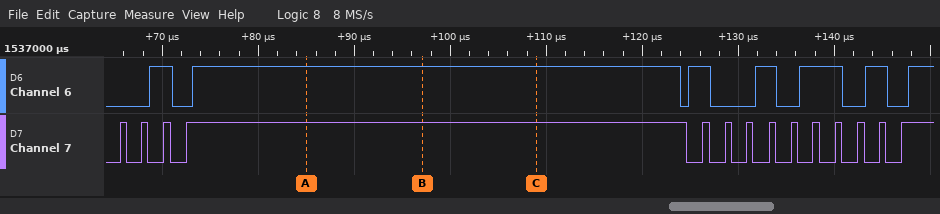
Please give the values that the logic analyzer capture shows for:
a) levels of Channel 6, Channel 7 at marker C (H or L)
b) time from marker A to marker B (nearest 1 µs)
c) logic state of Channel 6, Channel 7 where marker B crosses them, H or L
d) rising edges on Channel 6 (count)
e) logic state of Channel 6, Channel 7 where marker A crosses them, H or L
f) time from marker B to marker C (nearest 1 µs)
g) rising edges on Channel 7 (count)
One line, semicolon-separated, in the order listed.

Channel 6=H, Channel 7=H; 12 µs; Channel 6=H, Channel 7=H; 7; Channel 6=H, Channel 7=H; 12 µs; 14
